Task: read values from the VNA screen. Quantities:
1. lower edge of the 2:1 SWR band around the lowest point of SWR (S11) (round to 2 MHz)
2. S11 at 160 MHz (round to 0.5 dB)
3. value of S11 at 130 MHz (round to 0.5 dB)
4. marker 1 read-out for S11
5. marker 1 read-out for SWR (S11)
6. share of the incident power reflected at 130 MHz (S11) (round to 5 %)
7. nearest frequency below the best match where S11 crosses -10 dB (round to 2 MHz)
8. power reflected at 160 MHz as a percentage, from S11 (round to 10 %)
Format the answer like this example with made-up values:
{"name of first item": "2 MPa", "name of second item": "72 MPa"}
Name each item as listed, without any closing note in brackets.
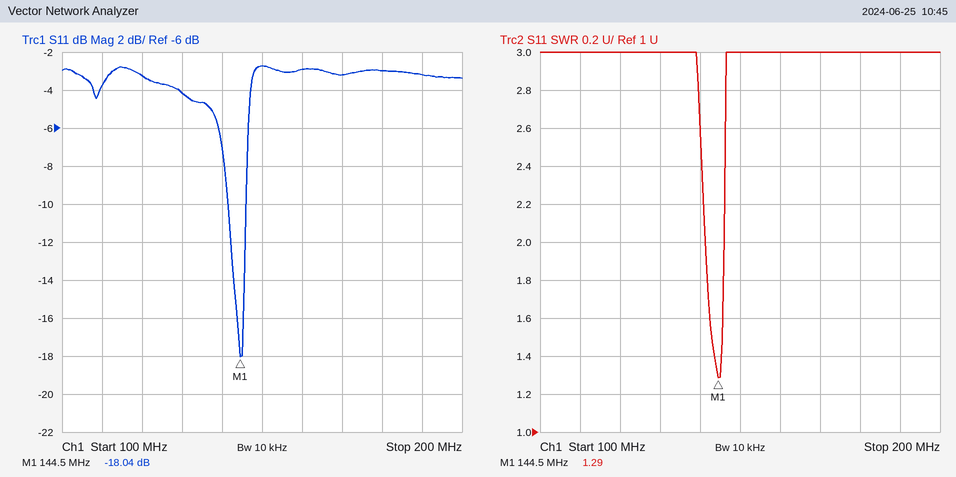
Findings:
{"lower edge of the 2:1 SWR band around the lowest point of SWR (S11)": "142 MHz", "S11 at 160 MHz": "-3.0 dB", "value of S11 at 130 MHz": "-4.0 dB", "marker 1 read-out for S11": "-18.04 dB", "marker 1 read-out for SWR": "1.29", "share of the incident power reflected at 130 MHz (S11)": "40 %", "nearest frequency below the best match where S11 crosses -10 dB": "142 MHz", "power reflected at 160 MHz as a percentage, from S11": "50 %"}
